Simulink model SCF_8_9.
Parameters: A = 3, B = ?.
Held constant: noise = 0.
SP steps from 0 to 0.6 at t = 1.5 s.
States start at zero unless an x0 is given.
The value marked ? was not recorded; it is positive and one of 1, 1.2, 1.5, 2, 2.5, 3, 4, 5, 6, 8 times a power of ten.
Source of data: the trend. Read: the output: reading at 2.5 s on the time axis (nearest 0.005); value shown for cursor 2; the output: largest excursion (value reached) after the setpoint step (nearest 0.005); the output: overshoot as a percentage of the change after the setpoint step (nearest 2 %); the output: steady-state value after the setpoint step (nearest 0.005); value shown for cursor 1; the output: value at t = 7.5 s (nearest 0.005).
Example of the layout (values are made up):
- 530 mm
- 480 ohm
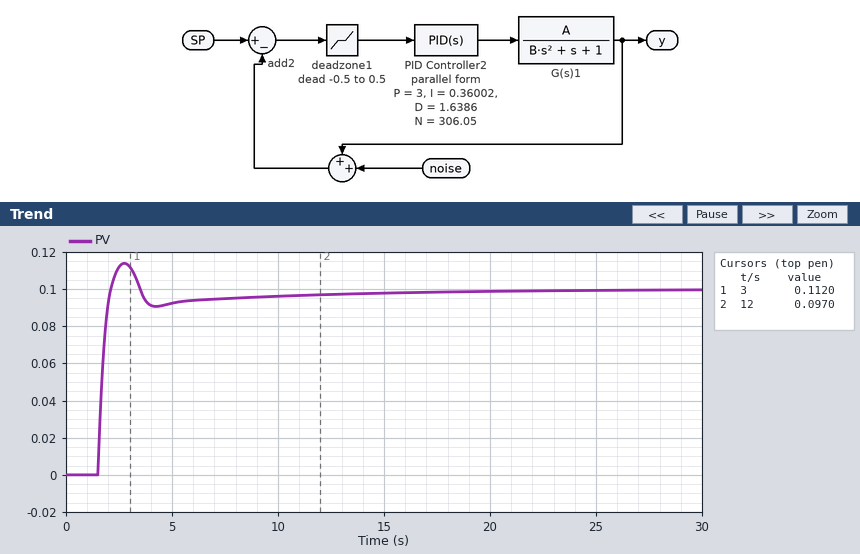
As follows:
- 0.110
- 0.0970
- 0.115
- 14 %
- 0.100
- 0.1120
- 0.095
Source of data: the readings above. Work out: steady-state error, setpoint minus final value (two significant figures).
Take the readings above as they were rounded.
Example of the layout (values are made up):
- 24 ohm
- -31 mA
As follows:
- 0.50
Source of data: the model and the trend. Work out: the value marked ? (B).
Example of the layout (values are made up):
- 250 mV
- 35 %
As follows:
- 1.5
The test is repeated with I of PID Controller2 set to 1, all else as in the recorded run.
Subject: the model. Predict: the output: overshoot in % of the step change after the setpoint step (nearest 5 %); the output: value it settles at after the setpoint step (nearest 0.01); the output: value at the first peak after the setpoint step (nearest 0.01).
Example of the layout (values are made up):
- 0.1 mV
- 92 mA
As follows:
- 30 %
- 0.10
- 0.13
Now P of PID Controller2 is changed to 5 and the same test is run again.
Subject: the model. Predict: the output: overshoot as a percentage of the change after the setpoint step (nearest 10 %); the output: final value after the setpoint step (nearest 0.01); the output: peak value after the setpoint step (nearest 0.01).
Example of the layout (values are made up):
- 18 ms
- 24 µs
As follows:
- 50 %
- 0.10
- 0.15
